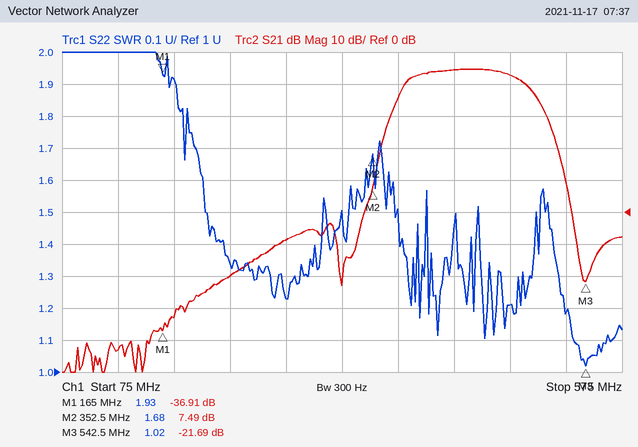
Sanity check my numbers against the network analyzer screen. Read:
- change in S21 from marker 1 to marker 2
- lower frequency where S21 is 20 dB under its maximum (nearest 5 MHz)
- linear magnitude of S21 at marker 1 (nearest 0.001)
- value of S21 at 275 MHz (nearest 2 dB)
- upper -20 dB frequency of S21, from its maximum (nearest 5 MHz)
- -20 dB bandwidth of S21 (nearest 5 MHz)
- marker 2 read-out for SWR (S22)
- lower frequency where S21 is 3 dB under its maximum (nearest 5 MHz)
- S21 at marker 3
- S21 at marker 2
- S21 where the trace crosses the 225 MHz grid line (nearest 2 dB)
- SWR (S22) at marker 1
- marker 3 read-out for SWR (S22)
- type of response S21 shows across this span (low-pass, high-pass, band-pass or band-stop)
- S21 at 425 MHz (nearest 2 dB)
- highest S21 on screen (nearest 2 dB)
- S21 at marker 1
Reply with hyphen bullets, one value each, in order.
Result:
- 44.40 dB
- 365 MHz
- 0.014
- -8 dB
- 515 MHz
- 150 MHz
- 1.68
- 385 MHz
- -21.69 dB
- 7.49 dB
- -20 dB
- 1.93
- 1.02
- band-pass
- 44 dB
- 44 dB
- -36.91 dB
